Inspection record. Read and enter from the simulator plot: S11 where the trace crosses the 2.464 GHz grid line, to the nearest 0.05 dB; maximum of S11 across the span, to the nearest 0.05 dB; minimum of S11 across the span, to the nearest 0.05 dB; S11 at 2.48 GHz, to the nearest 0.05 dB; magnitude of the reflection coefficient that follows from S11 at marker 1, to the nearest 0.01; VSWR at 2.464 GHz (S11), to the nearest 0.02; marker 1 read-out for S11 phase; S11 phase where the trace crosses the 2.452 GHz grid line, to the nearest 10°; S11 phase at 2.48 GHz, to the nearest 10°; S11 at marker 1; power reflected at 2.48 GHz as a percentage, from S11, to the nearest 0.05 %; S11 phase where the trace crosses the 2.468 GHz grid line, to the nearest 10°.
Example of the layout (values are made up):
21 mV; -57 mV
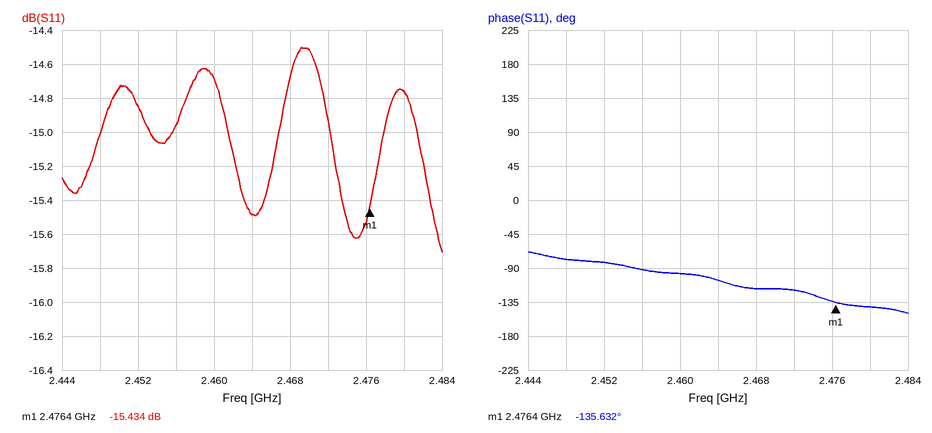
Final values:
-15.50 dB; -14.50 dB; -15.70 dB; -14.75 dB; 0.17; 1.40; -135.632°; -80°; -140°; -15.434 dB; 3.35 %; -120°
